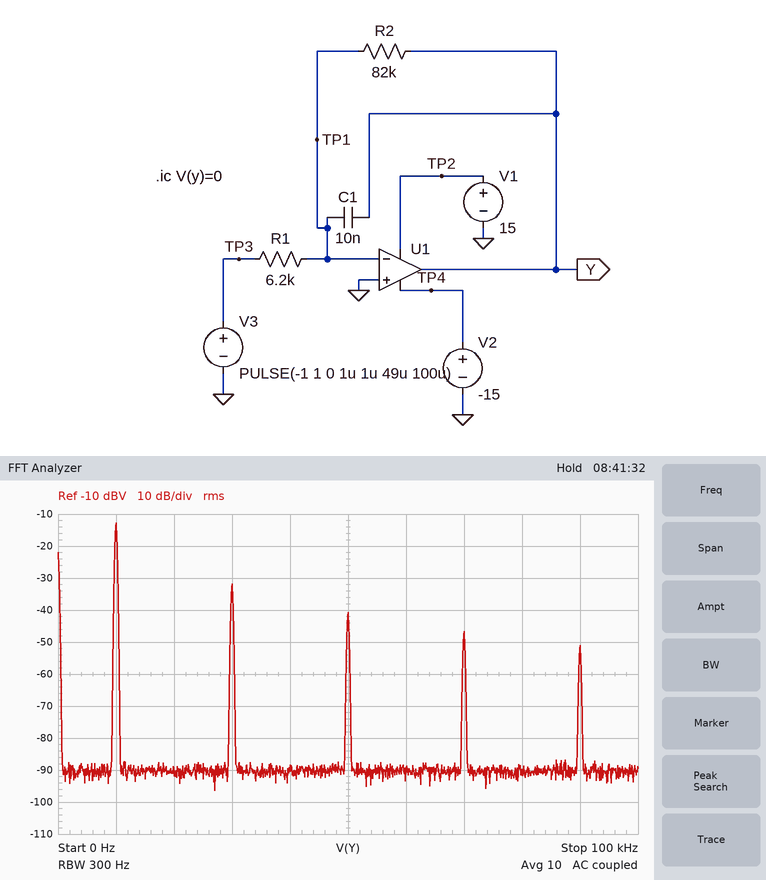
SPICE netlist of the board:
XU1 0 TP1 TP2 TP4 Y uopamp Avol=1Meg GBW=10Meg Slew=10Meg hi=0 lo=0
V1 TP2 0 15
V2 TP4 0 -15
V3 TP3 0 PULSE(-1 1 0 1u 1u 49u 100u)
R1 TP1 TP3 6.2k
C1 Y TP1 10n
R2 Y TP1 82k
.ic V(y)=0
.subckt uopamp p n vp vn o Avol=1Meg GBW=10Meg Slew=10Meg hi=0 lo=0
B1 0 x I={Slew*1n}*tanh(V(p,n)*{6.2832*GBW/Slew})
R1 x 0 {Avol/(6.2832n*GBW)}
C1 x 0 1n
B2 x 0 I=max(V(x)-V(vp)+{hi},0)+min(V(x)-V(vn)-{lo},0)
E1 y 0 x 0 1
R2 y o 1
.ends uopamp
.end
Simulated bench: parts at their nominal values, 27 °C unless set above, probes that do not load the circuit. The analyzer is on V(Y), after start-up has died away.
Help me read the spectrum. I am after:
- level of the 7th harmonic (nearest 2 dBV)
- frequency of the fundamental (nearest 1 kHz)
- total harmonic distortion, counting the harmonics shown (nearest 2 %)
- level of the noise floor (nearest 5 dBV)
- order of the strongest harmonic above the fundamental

-46 dBV
10 kHz
12 %
-90 dBV
3
